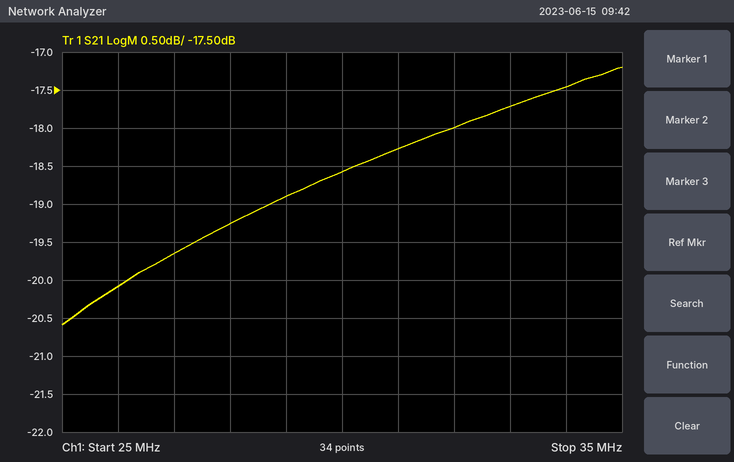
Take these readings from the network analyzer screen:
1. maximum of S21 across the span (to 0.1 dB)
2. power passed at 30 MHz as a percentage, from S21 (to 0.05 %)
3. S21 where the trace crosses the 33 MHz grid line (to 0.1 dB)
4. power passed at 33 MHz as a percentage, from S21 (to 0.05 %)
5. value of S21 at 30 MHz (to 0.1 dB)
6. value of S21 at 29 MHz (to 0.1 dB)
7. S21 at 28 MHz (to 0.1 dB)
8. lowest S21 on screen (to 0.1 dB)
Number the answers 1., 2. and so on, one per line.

1. -17.2 dB
2. 1.40 %
3. -17.7 dB
4. 1.70 %
5. -18.6 dB
6. -18.9 dB
7. -19.3 dB
8. -20.6 dB
